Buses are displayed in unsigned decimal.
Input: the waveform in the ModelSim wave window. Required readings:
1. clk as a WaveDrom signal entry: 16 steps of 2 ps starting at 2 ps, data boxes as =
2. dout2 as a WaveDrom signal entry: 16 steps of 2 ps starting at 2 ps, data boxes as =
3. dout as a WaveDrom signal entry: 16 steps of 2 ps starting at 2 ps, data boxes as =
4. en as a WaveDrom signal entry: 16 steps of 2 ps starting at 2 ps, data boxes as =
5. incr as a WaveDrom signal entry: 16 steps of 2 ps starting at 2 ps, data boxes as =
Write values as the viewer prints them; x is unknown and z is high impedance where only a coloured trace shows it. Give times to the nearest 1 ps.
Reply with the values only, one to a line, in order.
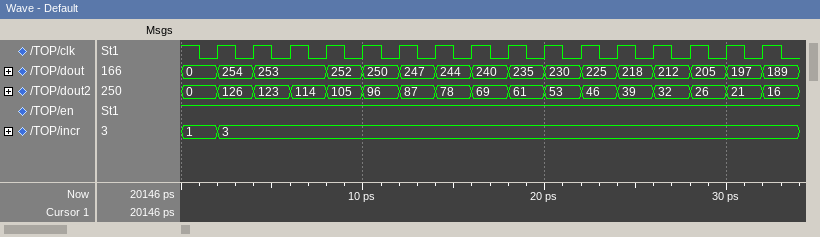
{name: 'clk', wave: 'p...............'}
{name: 'dout2', wave: '================', data: '126 123 114 105 96 87 78 69 61 53 46 39 32 26 21 16'}
{name: 'dout', wave: '==.=============', data: '254 253 252 250 247 244 240 235 230 225 218 212 205 197 189'}
{name: 'en', wave: '1...............'}
{name: 'incr', wave: '=...............', data: '3'}
